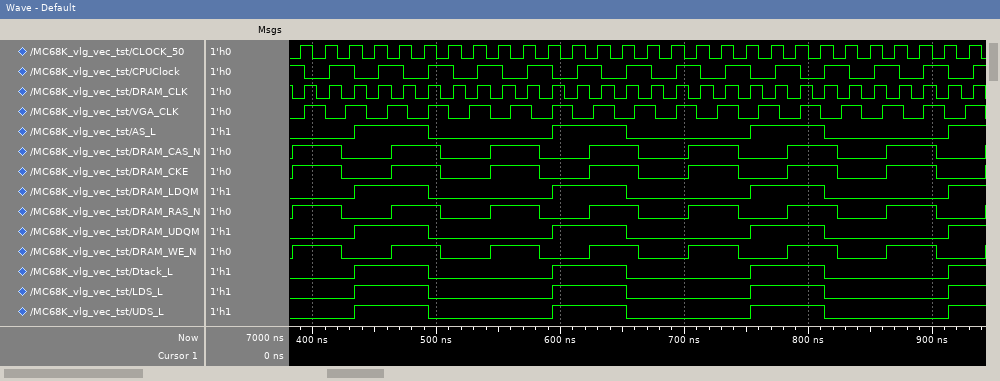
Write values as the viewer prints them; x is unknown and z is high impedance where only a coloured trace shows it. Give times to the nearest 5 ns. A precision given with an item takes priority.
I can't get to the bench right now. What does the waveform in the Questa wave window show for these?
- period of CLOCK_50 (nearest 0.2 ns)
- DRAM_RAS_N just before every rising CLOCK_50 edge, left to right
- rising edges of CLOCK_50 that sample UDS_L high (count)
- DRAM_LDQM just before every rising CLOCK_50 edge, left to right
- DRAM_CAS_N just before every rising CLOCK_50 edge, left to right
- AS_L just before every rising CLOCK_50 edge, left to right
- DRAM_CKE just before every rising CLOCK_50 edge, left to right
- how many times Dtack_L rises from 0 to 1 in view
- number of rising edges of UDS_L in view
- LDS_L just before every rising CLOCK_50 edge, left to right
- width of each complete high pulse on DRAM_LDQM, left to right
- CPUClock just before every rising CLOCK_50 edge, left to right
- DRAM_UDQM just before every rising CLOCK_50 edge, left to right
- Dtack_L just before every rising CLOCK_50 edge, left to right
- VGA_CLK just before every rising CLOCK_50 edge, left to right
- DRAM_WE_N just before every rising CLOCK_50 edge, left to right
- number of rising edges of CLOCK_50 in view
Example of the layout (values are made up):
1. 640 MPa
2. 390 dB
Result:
1. 20 ns
2. 1 1 0 0 1 1 0 0 1 1 0 0 1 1 0 0 1 1 0 0 1 1 0 0 1 1 0 0
3. 10
4. 0 0 0 1 1 1 0 0 0 0 0 1 1 1 0 0 0 0 0 1 1 1 0 0 0 0 0 1
5. 1 1 0 0 1 1 0 0 1 1 0 0 1 1 0 0 1 1 0 0 1 1 0 0 1 1 0 0
6. 0 0 0 1 1 1 0 0 0 0 0 1 1 1 0 0 0 0 0 1 1 1 0 0 0 0 0 1
7. 1 1 0 0 1 1 0 0 1 1 0 0 1 1 0 0 1 1 0 0 1 1 0 0 1 1 0 0
8. 4
9. 4
10. 0 0 0 1 1 1 0 0 0 0 0 1 1 1 0 0 0 0 0 1 1 1 0 0 0 0 0 1
11. 60 ns, 60 ns, 60 ns
12. 1 0 1 0 1 0 1 0 1 0 1 0 1 0 1 0 1 0 1 0 1 0 1 0 1 0 1 0
13. 0 0 0 1 1 1 0 0 0 0 0 1 1 1 0 0 0 0 0 1 1 1 0 0 0 0 0 1
14. 0 0 0 1 1 1 0 0 0 0 0 1 1 1 0 0 0 0 0 1 1 1 0 0 0 0 0 1
15. 0 1 1 0 1 0 1 1 0 1 0 1 1 0 1 0 1 1 0 1 0 1 1 0 1 0 1 1
16. 1 1 0 0 1 1 0 0 1 1 0 0 1 1 0 0 1 1 0 0 1 1 0 0 1 1 0 0
17. 28
